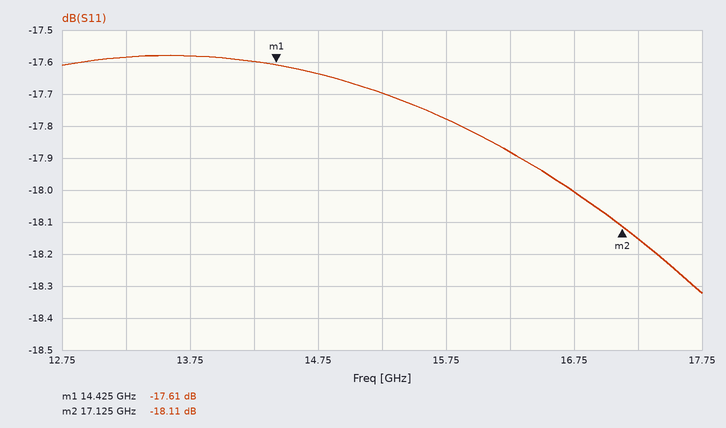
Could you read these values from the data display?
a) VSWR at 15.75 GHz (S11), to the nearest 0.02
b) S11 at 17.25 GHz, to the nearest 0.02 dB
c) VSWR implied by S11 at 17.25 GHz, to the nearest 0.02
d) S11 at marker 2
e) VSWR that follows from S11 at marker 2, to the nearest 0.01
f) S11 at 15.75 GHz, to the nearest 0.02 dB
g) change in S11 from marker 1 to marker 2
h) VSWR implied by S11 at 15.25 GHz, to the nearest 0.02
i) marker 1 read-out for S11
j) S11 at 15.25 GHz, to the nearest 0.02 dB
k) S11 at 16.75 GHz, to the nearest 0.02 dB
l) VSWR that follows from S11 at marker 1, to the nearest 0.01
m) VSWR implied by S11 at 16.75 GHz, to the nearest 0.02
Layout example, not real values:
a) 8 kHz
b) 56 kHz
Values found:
a) 1.30
b) -18.16 dB
c) 1.28
d) -18.11 dB
e) 1.28
f) -17.78 dB
g) -0.50 dB
h) 1.30
i) -17.61 dB
j) -17.70 dB
k) -18.00 dB
l) 1.30
m) 1.28
